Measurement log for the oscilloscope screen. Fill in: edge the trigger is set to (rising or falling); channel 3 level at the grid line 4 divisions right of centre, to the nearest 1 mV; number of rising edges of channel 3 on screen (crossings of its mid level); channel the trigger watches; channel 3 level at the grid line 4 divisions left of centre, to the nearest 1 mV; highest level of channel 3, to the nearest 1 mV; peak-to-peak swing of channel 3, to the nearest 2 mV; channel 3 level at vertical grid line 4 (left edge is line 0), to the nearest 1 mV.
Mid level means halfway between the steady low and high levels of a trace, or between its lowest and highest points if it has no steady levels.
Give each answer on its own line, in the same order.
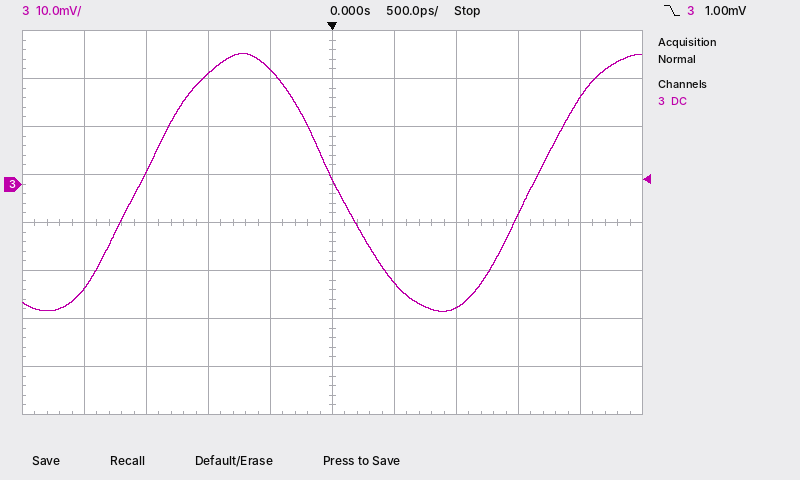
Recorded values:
falling
18 mV
2
channel 3
-22 mV
27 mV
54 mV
24 mV
